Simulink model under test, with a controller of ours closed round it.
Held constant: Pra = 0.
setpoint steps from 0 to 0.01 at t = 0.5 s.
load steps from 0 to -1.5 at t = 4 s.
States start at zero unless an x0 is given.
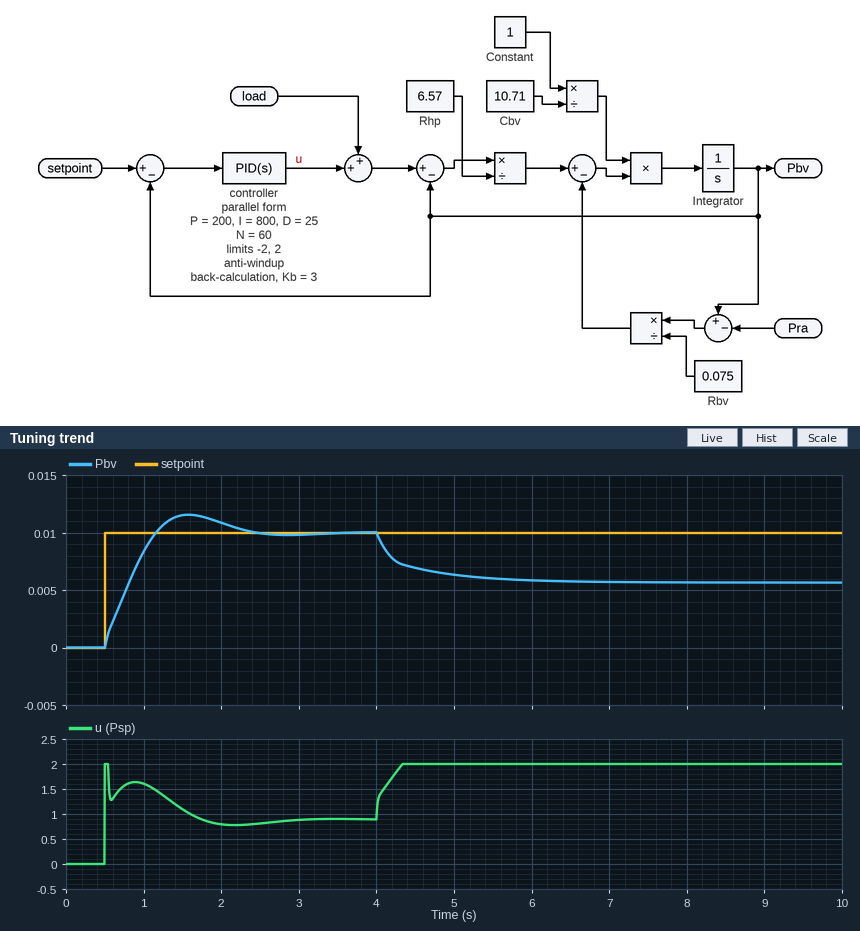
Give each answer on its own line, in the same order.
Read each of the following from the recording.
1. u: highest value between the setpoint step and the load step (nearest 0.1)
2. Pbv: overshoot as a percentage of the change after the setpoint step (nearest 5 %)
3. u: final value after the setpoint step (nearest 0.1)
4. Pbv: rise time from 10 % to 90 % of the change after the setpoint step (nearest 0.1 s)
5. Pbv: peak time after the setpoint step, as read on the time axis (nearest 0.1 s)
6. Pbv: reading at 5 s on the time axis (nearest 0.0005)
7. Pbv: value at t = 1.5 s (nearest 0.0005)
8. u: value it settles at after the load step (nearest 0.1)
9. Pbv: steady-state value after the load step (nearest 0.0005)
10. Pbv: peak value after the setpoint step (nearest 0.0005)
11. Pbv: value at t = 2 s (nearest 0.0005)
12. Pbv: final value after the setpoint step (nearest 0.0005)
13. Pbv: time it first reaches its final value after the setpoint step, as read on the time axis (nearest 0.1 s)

2.0
15 %
0.9
0.5 s
1.6 s
0.0065
0.0115
2.0
0.0055
0.0115
0.0110
0.0100
1.2 s
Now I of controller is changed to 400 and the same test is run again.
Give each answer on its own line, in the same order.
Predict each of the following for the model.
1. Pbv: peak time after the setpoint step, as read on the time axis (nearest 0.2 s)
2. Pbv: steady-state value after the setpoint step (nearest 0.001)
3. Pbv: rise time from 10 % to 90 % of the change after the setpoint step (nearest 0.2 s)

2.2 s
0.010
0.8 s
